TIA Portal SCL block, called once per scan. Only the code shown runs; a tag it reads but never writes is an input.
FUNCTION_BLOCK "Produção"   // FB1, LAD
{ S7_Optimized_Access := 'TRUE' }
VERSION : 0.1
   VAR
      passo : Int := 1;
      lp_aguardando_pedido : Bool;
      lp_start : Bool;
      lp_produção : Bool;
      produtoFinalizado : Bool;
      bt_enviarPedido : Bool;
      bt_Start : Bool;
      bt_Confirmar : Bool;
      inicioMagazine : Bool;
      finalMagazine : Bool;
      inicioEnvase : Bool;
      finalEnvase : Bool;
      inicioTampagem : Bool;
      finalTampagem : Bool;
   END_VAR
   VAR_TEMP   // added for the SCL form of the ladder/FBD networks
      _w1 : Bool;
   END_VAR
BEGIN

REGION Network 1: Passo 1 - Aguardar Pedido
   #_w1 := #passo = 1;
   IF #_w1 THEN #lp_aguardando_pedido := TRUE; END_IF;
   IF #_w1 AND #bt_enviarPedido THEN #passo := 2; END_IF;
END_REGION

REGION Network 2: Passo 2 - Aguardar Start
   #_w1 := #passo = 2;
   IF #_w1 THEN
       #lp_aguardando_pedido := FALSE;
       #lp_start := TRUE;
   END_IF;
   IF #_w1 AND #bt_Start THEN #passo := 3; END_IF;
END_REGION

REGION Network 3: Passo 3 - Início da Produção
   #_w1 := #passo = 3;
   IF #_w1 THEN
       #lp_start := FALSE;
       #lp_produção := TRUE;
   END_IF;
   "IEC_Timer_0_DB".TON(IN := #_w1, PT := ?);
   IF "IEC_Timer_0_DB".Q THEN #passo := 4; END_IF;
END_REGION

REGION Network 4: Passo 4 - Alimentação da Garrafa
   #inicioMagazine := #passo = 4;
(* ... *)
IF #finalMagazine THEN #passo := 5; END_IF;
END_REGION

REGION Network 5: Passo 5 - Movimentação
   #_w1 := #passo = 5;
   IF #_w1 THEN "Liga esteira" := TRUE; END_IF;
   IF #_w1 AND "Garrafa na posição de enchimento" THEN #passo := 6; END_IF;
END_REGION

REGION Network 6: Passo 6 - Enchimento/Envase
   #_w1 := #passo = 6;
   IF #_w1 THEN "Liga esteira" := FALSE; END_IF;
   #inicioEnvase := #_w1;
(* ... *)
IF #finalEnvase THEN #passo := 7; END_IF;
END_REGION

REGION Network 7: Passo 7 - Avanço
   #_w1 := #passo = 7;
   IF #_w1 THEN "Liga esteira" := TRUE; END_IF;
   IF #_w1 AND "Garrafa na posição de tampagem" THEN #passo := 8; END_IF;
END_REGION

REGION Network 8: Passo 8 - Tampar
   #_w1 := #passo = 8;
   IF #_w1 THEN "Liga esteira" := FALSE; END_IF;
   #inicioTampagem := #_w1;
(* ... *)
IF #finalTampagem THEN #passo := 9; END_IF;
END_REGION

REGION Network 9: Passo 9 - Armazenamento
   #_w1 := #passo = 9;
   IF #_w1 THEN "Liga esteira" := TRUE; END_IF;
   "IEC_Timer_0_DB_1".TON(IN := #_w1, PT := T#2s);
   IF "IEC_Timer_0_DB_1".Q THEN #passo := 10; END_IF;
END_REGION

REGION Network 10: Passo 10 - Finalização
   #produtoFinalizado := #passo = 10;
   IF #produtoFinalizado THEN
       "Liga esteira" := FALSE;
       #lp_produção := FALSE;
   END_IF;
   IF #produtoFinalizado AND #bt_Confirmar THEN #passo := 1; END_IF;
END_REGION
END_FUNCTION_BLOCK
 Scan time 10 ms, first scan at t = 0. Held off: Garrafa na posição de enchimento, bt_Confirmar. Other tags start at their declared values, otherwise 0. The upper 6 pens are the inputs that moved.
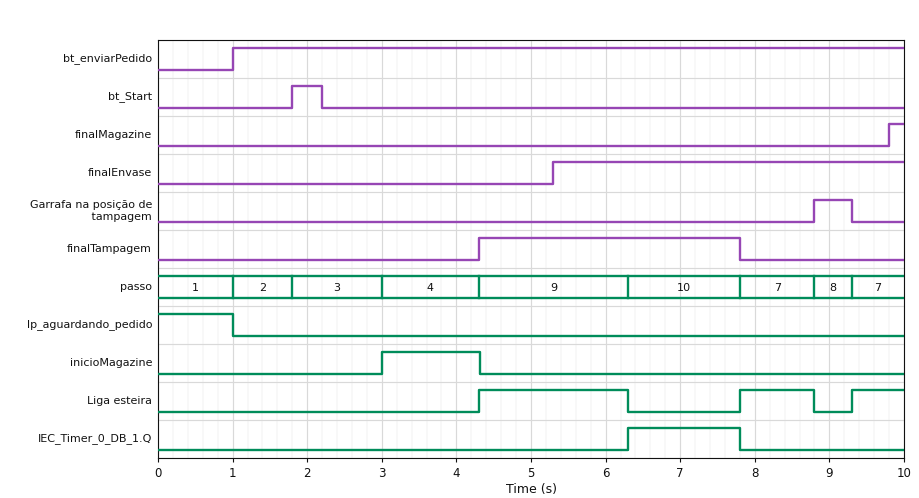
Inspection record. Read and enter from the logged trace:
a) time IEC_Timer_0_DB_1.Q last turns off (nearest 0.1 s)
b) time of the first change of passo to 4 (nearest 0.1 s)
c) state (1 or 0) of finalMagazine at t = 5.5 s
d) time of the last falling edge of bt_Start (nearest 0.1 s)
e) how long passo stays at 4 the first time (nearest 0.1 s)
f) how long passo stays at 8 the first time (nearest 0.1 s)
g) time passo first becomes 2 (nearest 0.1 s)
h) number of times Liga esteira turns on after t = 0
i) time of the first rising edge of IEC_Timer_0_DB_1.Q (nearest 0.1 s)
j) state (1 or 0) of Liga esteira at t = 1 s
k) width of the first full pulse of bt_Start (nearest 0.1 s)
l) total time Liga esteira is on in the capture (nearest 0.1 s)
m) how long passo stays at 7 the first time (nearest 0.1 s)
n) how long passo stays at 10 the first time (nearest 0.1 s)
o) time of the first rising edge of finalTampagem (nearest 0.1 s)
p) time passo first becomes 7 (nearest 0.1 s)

7.8 s
3.0 s
0
2.2 s
1.3 s
0.5 s
1.0 s
3
6.3 s
0
0.4 s
3.7 s
1.0 s
1.5 s
4.3 s
7.8 s
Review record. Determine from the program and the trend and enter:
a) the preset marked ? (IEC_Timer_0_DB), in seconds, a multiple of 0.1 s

1.2 s
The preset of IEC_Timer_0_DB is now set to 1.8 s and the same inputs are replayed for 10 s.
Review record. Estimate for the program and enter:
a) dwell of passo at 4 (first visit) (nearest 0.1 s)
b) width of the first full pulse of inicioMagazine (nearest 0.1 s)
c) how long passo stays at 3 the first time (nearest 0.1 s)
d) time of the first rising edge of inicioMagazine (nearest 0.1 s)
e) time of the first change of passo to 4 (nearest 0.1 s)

0.7 s
0.7 s
1.8 s
3.6 s
3.6 s
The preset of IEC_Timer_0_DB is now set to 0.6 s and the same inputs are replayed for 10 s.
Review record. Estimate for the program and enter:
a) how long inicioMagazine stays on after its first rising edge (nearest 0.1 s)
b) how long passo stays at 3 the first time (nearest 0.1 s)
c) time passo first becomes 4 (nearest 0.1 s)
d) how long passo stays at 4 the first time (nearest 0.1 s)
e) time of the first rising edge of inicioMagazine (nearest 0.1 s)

1.9 s
0.6 s
2.4 s
1.9 s
2.4 s
